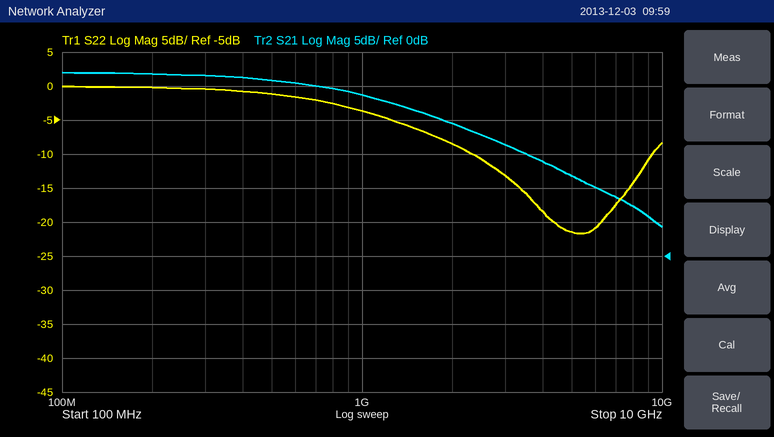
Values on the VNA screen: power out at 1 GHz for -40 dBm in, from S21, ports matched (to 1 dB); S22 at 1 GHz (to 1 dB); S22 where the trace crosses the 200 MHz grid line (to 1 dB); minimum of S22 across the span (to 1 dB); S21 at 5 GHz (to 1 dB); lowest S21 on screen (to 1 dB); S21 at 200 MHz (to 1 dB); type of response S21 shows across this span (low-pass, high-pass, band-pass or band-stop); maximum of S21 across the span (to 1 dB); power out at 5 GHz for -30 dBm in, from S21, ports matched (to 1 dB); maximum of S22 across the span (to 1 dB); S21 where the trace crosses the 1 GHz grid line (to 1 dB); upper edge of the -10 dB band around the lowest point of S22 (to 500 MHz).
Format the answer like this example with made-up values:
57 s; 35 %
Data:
-16 dBm; -4 dB; 0 dB; -22 dB; 12 dB; 4 dB; 27 dB; low-pass; 27 dB; -18 dBm; 0 dB; 24 dB; 9.5 GHz
